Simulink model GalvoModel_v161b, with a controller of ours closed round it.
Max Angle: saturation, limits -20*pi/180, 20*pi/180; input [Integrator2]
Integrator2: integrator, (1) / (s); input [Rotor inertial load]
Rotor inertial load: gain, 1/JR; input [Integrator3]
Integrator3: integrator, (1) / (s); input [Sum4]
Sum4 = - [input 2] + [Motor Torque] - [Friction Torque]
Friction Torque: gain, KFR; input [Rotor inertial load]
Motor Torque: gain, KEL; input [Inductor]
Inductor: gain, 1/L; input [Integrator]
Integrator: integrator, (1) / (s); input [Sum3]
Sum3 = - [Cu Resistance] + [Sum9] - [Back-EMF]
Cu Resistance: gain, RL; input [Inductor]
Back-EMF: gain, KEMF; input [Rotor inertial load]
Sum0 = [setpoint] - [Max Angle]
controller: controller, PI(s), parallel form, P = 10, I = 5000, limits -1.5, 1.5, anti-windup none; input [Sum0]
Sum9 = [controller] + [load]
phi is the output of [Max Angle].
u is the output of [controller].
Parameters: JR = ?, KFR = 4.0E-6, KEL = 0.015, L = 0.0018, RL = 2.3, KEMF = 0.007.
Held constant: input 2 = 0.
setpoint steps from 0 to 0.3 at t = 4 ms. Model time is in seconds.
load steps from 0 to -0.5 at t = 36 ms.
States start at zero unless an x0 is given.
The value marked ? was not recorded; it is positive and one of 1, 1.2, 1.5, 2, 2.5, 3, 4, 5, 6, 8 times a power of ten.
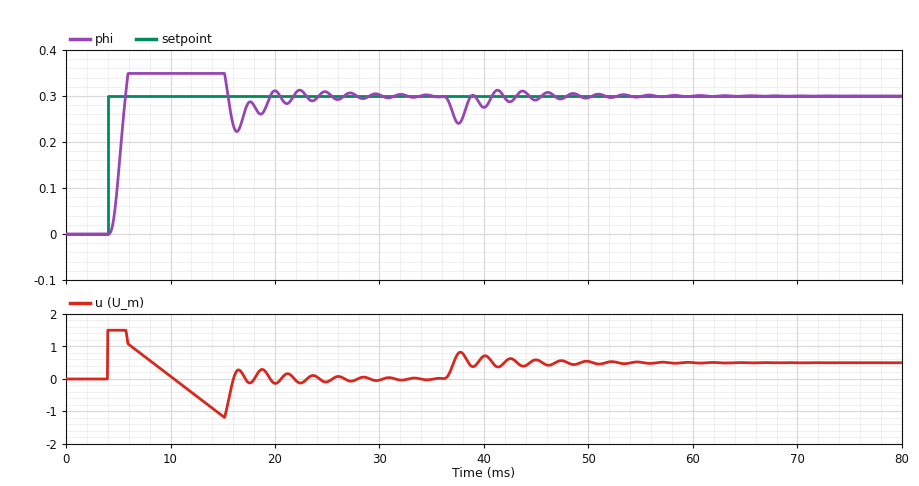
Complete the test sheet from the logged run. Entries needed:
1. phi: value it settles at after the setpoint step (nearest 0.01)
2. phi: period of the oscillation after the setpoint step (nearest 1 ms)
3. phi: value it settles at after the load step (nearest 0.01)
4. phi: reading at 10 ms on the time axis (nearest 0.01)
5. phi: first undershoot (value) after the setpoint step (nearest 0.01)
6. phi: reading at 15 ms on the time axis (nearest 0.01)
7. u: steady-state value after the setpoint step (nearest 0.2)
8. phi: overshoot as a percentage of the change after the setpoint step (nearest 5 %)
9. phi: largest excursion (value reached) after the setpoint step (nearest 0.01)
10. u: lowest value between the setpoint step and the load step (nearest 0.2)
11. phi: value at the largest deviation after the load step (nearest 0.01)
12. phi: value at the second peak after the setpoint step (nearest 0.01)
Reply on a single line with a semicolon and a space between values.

0.30; 7 ms; 0.30; 0.35; 0.22; 0.35; 0.0; 15 %; 0.35; -1.2; 0.24; 0.29
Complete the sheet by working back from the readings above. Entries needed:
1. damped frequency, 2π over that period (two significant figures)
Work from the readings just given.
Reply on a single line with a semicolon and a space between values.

0.90 rad/ms
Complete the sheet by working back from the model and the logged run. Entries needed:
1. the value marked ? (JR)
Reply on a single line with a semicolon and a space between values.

8e-09
